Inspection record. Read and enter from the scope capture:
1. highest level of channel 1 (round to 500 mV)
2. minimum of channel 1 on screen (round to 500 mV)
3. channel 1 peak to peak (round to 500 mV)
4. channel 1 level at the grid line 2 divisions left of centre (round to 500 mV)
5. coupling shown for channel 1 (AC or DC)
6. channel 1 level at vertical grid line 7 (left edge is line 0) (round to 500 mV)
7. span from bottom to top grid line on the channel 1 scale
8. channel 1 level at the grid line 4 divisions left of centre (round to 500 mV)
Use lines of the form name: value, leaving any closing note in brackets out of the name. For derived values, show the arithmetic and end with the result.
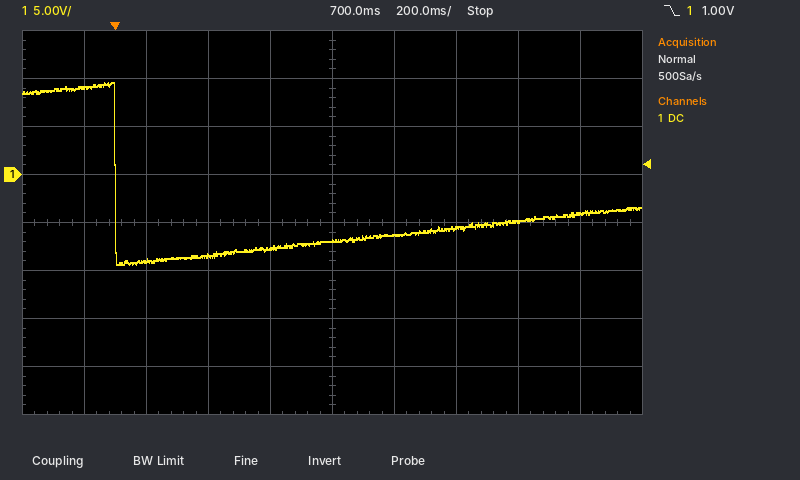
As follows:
highest level of channel 1: 9.5 V
minimum of channel 1 on screen: -9.5 V
channel 1 peak to peak: 9.5 V − (-9.5 V) = 19.0 V
channel 1 level at the grid line 2 divisions left of centre: -8.5 V
coupling shown for channel 1: DC
channel 1 level at vertical grid line 7 (left edge is line 0): -5.5 V
span from bottom to top grid line on the channel 1 scale: 40 V
channel 1 level at the grid line 4 divisions left of centre: 9.0 V
